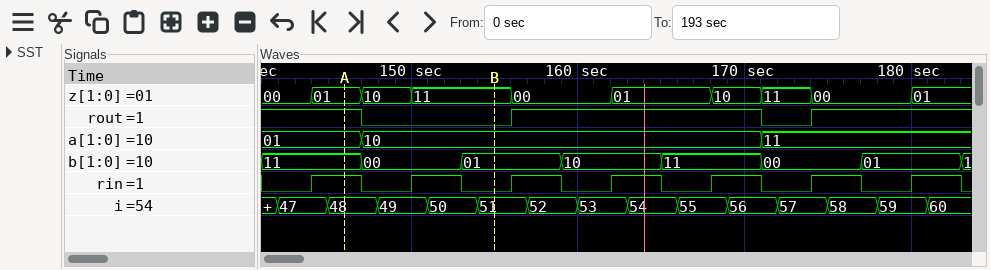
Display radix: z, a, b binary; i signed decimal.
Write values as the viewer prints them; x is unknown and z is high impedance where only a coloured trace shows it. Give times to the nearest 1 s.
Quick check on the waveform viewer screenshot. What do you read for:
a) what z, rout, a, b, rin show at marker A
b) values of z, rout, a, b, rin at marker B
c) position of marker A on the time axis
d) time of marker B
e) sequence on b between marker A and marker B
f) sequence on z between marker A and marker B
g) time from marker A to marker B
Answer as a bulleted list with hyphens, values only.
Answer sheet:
- z=01, rout=1, a=01, b=11, rin=1
- z=11, rout=0, a=10, b=01, rin=0
- 146 s
- 155 s
- 11, 00, 01
- 01, 10, 11
- 9 s
